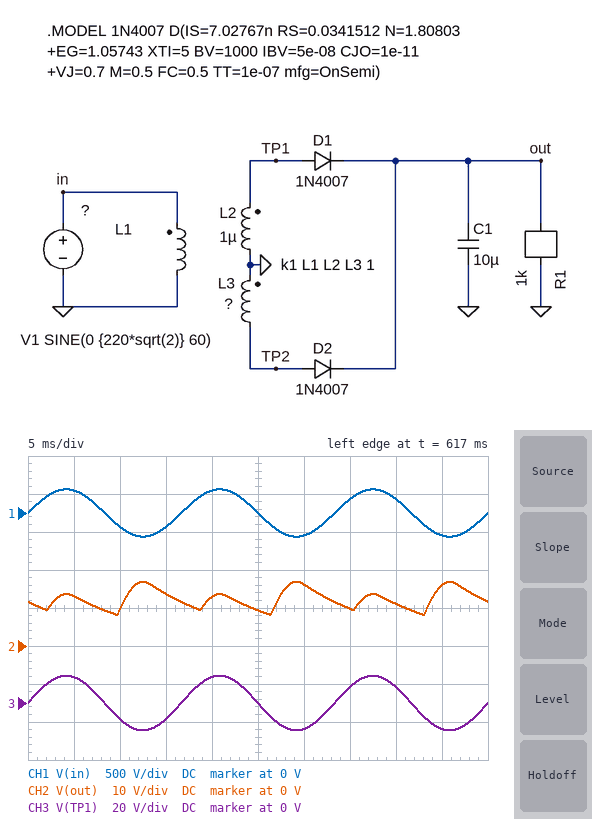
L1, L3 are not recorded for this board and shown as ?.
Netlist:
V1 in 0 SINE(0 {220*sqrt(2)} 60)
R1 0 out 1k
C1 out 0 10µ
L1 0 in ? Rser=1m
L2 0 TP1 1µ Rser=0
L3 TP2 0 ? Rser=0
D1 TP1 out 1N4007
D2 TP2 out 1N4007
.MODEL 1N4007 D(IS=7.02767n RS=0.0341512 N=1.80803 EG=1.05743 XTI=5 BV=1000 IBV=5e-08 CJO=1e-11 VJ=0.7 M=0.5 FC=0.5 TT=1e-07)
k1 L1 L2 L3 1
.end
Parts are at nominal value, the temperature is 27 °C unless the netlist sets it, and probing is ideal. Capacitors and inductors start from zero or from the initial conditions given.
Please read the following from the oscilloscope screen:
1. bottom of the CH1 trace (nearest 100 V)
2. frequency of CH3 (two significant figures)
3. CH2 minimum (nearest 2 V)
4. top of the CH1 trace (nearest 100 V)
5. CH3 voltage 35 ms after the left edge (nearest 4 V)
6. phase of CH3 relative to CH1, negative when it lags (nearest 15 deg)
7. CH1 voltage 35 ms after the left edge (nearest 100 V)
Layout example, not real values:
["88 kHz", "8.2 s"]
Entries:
["-300 V", "60 Hz", "8 V", "300 V", "8 V", "0 deg", "200 V"]
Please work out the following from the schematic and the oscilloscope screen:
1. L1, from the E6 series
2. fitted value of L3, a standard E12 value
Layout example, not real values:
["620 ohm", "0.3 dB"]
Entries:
["470 µH", "1.5 µH"]
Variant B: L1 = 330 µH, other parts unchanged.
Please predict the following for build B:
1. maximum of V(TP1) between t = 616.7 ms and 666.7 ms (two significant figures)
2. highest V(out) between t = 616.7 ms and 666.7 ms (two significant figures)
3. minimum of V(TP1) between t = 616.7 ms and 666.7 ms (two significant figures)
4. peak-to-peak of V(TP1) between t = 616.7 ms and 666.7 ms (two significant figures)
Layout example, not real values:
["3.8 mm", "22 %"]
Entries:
["17 V", "20 V", "-17 V", "34 V"]
